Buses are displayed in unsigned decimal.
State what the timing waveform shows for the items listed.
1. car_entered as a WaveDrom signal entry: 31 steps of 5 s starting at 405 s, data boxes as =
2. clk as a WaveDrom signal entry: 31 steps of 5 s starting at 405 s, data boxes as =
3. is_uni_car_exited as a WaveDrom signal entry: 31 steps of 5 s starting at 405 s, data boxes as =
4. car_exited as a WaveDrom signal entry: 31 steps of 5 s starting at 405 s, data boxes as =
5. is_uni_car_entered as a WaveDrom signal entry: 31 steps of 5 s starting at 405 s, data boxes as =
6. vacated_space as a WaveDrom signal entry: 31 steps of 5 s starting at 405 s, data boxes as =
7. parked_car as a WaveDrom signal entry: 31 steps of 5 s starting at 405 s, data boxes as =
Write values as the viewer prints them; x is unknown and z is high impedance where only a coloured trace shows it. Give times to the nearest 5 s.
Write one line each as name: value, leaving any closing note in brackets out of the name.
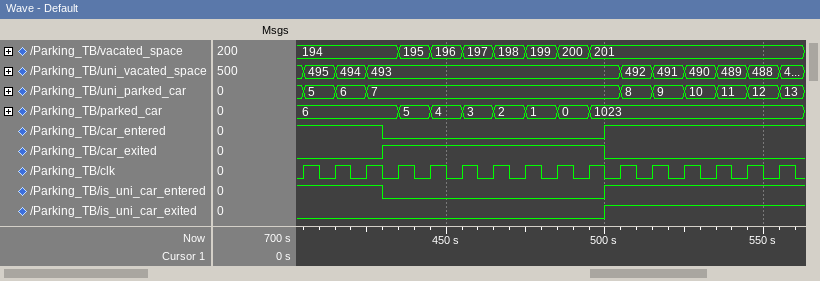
car_entered as a WaveDrom signal entry: 31 steps of 5 s starting at 405 s, data boxes as =: {name: 'car_entered', wave: '1....0.............1...........'}
clk as a WaveDrom signal entry: 31 steps of 5 s starting at 405 s, data boxes as =: {name: 'clk', wave: '1010101010101010101010101010101'}
is_uni_car_exited as a WaveDrom signal entry: 31 steps of 5 s starting at 405 s, data boxes as =: {name: 'is_uni_car_exited', wave: '0..................1...........'}
car_exited as a WaveDrom signal entry: 31 steps of 5 s starting at 405 s, data boxes as =: {name: 'car_exited', wave: '0....1.............0...........'}
is_uni_car_entered as a WaveDrom signal entry: 31 steps of 5 s starting at 405 s, data boxes as =: {name: 'is_uni_car_entered', wave: '1....0.............1...........'}
vacated_space as a WaveDrom signal entry: 31 steps of 5 s starting at 405 s, data boxes as =: {name: 'vacated_space', wave: '=.....=.=.=.=.=.=.=............', data: '194 195 196 197 198 199 200 201'}
parked_car as a WaveDrom signal entry: 31 steps of 5 s starting at 405 s, data boxes as =: {name: 'parked_car', wave: '=.....=.=.=.=.=.=.=............', data: '6 5 4 3 2 1 0 1023'}
